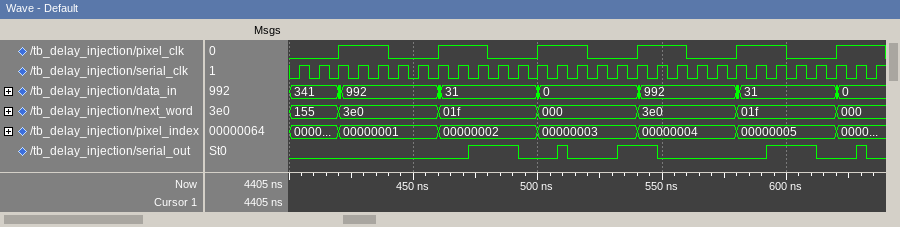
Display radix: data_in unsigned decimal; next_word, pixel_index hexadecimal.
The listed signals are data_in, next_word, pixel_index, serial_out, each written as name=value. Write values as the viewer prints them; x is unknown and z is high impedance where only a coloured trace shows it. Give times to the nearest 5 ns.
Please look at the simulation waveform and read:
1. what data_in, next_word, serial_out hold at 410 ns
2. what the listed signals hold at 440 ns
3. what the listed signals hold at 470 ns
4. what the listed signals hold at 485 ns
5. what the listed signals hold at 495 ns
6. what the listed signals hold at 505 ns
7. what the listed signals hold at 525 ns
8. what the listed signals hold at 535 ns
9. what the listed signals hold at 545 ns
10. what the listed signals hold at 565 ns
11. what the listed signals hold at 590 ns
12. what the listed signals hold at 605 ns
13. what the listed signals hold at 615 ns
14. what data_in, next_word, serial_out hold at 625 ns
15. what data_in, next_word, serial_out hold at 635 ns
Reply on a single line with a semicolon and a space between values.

data_in=341, next_word=155, serial_out=0; data_in=992, next_word=3e0, pixel_index=00000001, serial_out=0; data_in=31, next_word=01f, pixel_index=00000002, serial_out=0; data_in=31, next_word=01f, pixel_index=00000002, serial_out=1; data_in=31, next_word=01f, pixel_index=00000002, serial_out=0; data_in=0, next_word=000, pixel_index=00000003, serial_out=0; data_in=0, next_word=000, pixel_index=00000003, serial_out=0; data_in=0, next_word=000, pixel_index=00000003, serial_out=1; data_in=992, next_word=3e0, pixel_index=00000004, serial_out=1; data_in=992, next_word=3e0, pixel_index=00000004, serial_out=0; data_in=31, next_word=01f, pixel_index=00000005, serial_out=0; data_in=31, next_word=01f, pixel_index=00000005, serial_out=1; data_in=31, next_word=01f, pixel_index=00000005, serial_out=0; data_in=0, next_word=000, serial_out=0; data_in=0, next_word=000, serial_out=0
